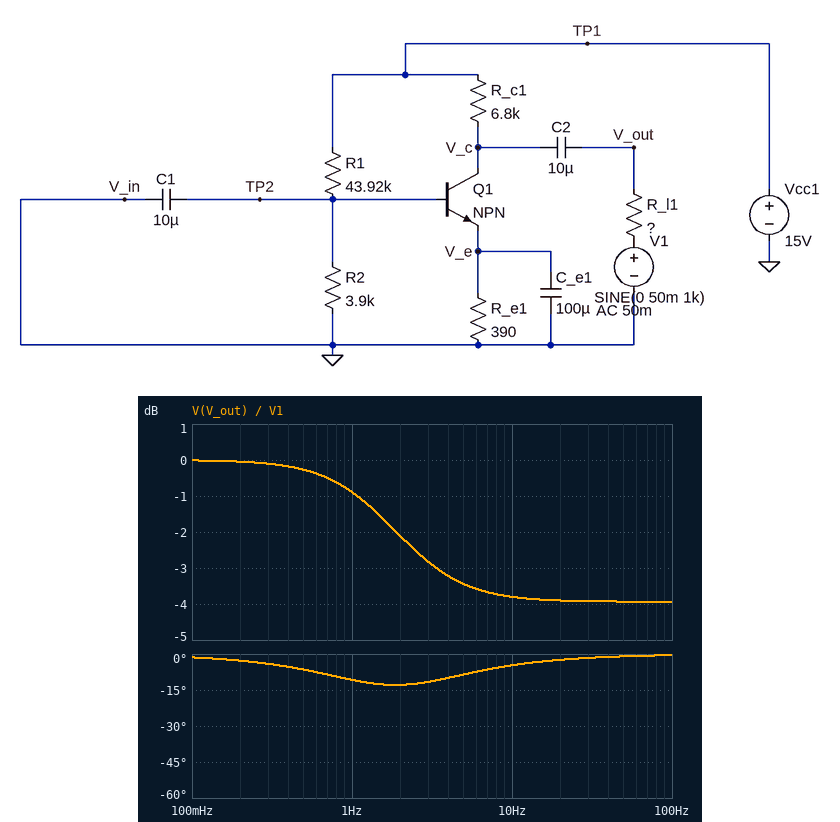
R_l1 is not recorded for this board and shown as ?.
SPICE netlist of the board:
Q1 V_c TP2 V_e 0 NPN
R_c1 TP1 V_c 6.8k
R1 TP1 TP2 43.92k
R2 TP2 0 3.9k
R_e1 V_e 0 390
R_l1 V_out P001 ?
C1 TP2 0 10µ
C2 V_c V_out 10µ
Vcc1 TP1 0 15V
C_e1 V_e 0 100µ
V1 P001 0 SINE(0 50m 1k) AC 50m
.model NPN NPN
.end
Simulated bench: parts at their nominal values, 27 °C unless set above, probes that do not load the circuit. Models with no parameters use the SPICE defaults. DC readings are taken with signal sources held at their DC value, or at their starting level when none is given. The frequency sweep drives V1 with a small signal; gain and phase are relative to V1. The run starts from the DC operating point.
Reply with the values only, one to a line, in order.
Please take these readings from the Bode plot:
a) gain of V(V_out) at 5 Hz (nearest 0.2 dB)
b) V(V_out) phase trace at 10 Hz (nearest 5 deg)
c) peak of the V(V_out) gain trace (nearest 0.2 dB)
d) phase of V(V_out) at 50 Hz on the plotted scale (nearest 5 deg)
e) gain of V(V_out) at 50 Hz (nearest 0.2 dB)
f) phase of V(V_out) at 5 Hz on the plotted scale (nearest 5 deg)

-3.4 dB
-5 deg
0 dB
0 deg
-4.0 dB
-10 deg
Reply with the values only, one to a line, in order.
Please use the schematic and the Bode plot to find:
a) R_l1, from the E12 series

3.9 kΩ
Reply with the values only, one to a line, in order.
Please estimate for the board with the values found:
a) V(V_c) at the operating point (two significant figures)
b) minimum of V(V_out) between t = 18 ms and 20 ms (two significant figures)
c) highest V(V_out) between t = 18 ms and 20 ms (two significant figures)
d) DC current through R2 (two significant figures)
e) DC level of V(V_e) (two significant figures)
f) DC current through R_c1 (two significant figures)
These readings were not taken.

7.9 V
-32 mV
32 mV
300 µA
410 mV
1.0 mA
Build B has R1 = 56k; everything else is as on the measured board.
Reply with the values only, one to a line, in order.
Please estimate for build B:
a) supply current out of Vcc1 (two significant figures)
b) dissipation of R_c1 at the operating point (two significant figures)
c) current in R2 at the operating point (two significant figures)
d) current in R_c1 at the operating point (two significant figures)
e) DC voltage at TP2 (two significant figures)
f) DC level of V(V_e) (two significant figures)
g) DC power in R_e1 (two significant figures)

760 µA
1.8 mW
250 µA
510 µA
960 mV
200 mV
100 µW
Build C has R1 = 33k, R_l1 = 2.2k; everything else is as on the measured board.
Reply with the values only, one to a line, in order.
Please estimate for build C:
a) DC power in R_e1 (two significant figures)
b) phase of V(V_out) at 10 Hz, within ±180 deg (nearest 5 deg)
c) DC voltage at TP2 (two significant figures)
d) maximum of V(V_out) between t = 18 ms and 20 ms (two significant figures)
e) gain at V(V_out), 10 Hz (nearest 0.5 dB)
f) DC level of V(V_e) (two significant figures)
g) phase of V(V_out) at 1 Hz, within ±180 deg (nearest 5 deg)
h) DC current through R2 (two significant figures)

1.4 mW
-5 deg
1.5 V
38 mV
-2.5 dB
730 mV
-5 deg
390 µA
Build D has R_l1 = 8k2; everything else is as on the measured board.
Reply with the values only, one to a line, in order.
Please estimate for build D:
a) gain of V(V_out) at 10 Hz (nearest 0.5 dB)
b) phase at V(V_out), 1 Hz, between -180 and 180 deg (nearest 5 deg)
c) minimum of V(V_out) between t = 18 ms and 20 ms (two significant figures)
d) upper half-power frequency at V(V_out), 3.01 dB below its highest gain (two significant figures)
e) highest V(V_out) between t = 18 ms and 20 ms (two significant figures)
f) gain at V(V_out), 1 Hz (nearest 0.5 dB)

-6.5 dB
-20 deg
-23 mV
1.4 Hz
23 mV
-2.0 dB
